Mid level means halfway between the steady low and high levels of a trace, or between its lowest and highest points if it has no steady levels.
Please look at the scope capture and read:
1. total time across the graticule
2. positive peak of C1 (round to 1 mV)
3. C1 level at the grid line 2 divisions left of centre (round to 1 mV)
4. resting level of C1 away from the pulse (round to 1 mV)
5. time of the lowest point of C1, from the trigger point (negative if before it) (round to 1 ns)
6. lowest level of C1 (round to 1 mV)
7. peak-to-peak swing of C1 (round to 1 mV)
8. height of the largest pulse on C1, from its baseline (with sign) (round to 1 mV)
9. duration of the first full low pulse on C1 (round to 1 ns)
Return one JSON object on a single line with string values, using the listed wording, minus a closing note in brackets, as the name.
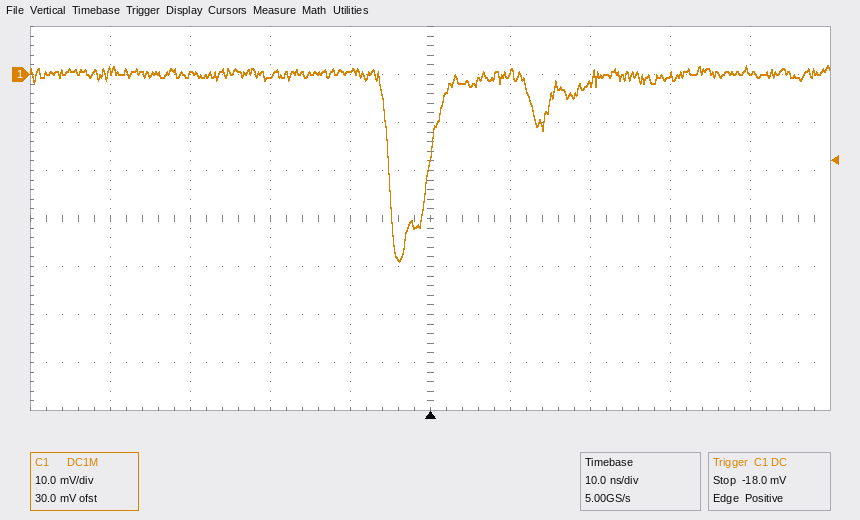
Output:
{"total time across the graticule": "100 ns", "positive peak of C1": "2 mV", "C1 level at the grid line 2 divisions left of centre": "0 mV", "resting level of C1 away from the pulse": "0 mV", "time of the lowest point of C1, from the trigger point (negative if before it)": "-4 ns", "lowest level of C1": "-39 mV", "peak-to-peak swing of C1": "41 mV", "height of the largest pulse on C1, from its baseline (with sign)": "-39 mV", "duration of the first full low pulse on C1": "5 ns"}
